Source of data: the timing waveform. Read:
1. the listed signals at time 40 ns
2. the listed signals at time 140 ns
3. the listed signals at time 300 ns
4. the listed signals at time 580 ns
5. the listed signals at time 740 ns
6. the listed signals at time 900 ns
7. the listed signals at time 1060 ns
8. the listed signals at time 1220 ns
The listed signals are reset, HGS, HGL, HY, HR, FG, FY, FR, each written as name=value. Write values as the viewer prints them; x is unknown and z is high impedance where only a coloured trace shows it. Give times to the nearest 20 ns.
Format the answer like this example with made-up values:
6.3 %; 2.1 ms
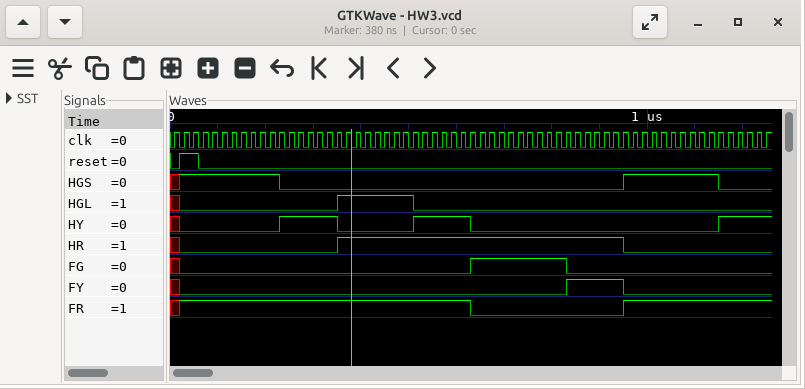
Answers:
reset=1, HGS=1, HGL=0, HY=0, HR=0, FG=0, FY=0, FR=1; reset=0, HGS=1, HGL=0, HY=0, HR=0, FG=0, FY=0, FR=1; reset=0, HGS=0, HGL=0, HY=1, HR=0, FG=0, FY=0, FR=1; reset=0, HGS=0, HGL=0, HY=1, HR=1, FG=0, FY=0, FR=1; reset=0, HGS=0, HGL=0, HY=0, HR=1, FG=1, FY=0, FR=0; reset=0, HGS=0, HGL=0, HY=0, HR=1, FG=0, FY=1, FR=0; reset=0, HGS=1, HGL=0, HY=0, HR=0, FG=0, FY=0, FR=1; reset=0, HGS=0, HGL=0, HY=1, HR=0, FG=0, FY=0, FR=1
